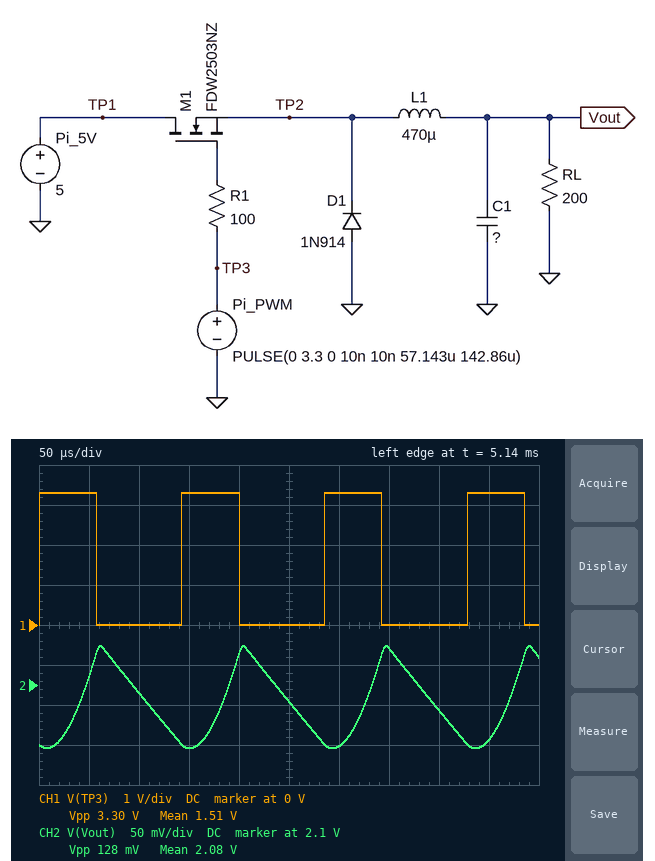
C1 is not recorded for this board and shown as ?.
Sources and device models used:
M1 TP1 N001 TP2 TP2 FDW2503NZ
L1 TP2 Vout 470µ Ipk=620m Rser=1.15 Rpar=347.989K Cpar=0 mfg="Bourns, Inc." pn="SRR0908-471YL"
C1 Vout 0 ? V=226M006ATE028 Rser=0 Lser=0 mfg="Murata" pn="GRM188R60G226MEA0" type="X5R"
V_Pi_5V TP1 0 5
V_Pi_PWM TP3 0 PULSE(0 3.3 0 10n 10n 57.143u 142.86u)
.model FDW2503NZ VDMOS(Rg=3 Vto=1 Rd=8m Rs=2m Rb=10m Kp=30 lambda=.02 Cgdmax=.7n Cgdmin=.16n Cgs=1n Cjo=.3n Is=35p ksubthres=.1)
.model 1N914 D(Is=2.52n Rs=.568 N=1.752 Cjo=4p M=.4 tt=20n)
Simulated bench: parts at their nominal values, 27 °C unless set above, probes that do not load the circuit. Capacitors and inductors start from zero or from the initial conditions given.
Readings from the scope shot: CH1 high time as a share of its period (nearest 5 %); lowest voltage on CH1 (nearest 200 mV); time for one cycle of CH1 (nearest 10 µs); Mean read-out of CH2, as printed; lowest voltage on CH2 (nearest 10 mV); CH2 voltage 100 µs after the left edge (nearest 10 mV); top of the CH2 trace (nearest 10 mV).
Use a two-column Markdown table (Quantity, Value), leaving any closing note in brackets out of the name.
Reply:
| Quantity | Value |
|---|---|
| CH1 high time as a share of its period | 40 % |
| lowest voltage on CH1 | 0 V |
| time for one cycle of CH1 | 140 µs |
| Mean read-out of CH2, as printed | 2.08 V |
| lowest voltage on CH2 | 2.02 V |
| CH2 voltage 100 µs after the left edge | 2.09 V |
| top of the CH2 trace | 2.15 V |
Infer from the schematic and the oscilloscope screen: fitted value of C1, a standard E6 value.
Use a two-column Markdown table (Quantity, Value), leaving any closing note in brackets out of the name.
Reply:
| Quantity | Value |
|---|---|
| fitted value of C1, a standard E6 value | 6.8 µF |
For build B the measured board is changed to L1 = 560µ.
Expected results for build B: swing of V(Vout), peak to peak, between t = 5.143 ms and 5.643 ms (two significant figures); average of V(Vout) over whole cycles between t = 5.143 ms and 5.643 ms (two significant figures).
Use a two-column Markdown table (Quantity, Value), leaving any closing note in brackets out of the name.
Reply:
| Quantity | Value |
|---|---|
| swing of V(Vout), peak to peak, between t = 5.143 ms and 5.643 ms | 120 mV |
| average of V(Vout) over whole cycles between t = 5.143 ms and 5.643 ms | 2.0 V |
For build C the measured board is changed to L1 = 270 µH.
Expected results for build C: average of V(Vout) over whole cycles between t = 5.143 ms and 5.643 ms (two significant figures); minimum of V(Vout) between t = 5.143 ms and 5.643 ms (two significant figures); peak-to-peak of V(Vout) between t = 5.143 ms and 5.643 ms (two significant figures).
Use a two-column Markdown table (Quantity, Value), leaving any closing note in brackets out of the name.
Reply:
| Quantity | Value |
|---|---|
| average of V(Vout) over whole cycles between t = 5.143 ms and 5.643 ms | 2.2 V |
| minimum of V(Vout) between t = 5.143 ms and 5.643 ms | 2.1 V |
| peak-to-peak of V(Vout) between t = 5.143 ms and 5.643 ms | 140 mV |
